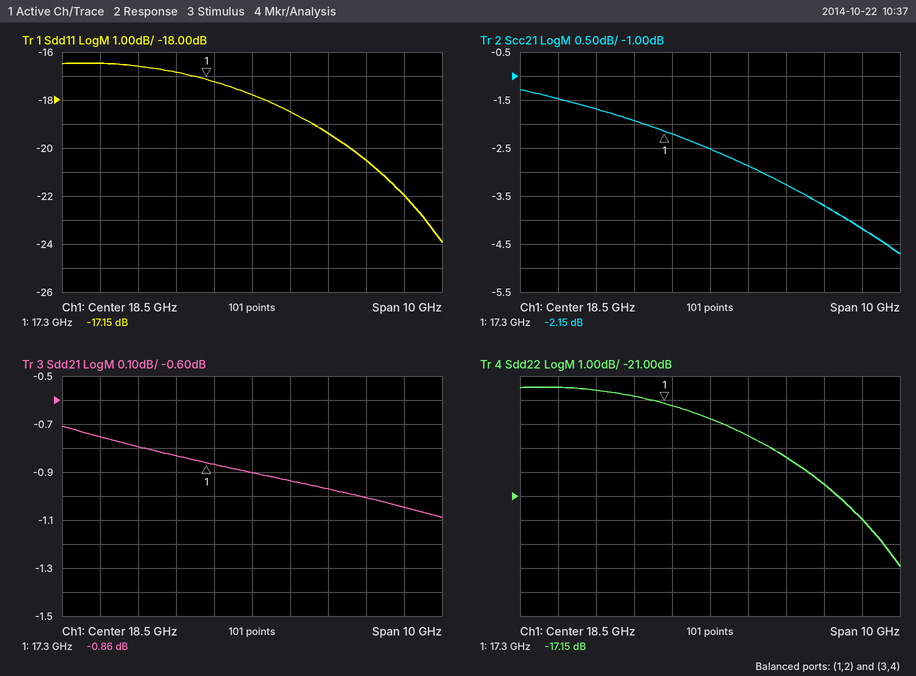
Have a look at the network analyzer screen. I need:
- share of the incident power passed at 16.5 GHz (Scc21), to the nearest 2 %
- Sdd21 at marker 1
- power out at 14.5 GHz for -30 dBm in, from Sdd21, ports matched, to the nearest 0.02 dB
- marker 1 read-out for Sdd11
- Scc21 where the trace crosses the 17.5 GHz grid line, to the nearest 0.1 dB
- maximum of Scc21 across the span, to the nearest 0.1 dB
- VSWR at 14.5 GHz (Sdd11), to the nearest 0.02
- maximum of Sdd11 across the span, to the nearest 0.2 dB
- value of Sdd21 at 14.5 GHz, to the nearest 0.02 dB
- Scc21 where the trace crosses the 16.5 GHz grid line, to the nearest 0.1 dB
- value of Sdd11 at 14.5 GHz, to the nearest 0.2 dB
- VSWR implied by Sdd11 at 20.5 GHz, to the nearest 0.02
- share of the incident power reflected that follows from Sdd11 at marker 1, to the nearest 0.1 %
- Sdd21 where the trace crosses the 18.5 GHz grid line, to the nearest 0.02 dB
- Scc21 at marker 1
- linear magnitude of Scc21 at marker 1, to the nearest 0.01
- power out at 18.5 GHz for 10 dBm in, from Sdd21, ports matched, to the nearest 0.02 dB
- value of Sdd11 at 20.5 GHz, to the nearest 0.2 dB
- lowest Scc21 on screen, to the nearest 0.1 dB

64 %
-0.86 dB
-30.76 dBm
-17.15 dB
-2.2 dB
-1.3 dB
1.36
-16.4 dB
-0.76 dB
-1.9 dB
-16.4 dB
1.24
1.9 %
-0.90 dB
-2.15 dB
0.78
9.10 dBm
-19.4 dB
-4.7 dB
